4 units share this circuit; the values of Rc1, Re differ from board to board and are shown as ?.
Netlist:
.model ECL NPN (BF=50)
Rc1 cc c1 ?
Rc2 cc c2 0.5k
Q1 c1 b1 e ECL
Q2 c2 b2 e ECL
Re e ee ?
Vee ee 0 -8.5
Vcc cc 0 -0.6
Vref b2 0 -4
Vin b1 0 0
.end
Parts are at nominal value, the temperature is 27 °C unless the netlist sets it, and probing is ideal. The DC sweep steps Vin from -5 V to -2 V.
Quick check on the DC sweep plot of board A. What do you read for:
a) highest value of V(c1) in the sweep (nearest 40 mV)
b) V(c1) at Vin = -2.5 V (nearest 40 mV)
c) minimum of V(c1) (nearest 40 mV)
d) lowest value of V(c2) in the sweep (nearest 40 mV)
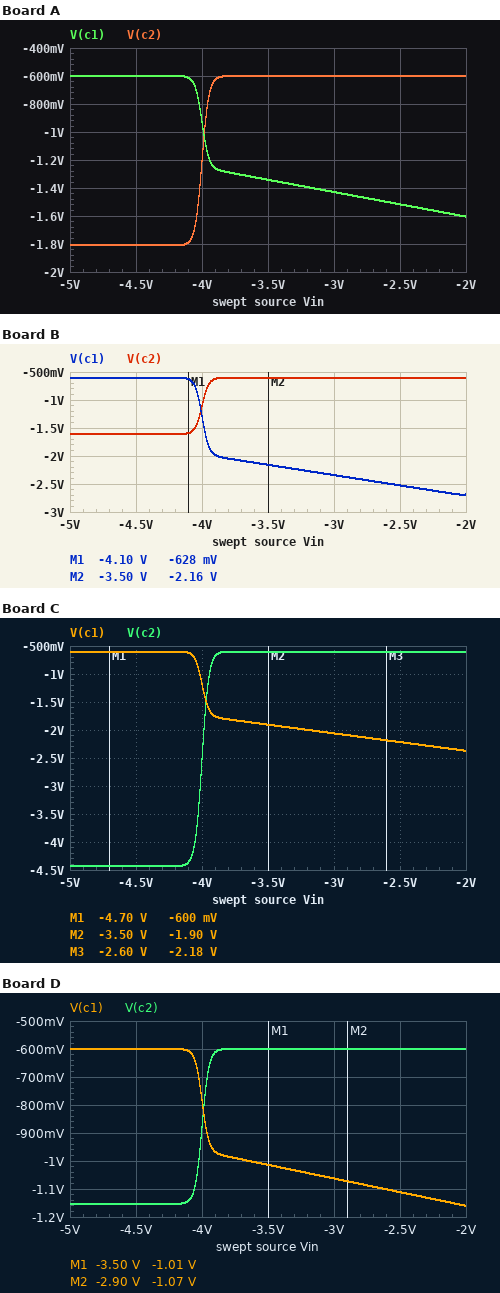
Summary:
-600 mV
-1.52 V
-1.60 V
-1.80 V
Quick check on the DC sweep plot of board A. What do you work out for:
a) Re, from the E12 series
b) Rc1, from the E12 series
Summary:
1.5 kΩ
270 Ω
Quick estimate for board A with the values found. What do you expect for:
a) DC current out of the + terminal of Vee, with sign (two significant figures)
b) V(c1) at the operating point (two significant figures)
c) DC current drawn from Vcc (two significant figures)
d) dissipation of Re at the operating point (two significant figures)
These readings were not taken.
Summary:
-5.1 mA
-810 mV
780 µA
39 mW
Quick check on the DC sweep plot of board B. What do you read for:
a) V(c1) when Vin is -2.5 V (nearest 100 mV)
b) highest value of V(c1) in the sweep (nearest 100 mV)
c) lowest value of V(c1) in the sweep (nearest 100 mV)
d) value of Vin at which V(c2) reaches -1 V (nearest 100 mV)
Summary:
-2.5 V
-600 mV
-2.7 V
-4.0 V
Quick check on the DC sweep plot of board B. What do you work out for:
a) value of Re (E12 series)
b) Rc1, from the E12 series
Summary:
1.8 kΩ
680 Ω
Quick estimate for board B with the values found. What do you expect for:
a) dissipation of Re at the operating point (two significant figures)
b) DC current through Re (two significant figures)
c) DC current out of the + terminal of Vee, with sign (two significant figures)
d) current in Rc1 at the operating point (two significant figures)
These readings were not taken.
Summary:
33 mW
4.3 mA
-4.3 mA
310 µA
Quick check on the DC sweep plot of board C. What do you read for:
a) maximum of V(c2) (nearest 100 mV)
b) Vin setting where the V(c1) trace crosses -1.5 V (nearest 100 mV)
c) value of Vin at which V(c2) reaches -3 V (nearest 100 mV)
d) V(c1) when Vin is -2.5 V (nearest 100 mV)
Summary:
-600 mV
-4.0 V
-4.0 V
-2.2 V
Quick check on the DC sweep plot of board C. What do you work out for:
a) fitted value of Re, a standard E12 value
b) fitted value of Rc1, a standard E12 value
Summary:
470 Ω
150 Ω
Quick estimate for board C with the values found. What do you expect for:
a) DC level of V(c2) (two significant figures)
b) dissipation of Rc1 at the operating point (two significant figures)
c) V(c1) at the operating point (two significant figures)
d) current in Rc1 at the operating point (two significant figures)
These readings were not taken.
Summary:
-600 mV
390 µW
-840 mV
1.6 mA
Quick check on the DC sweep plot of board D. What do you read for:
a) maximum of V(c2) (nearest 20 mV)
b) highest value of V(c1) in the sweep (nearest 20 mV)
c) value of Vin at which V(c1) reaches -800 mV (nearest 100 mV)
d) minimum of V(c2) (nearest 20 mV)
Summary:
-600 mV
-600 mV
-4.0 V
-1.16 V
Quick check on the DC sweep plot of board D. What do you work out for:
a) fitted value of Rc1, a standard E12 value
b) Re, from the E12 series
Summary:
330 Ω
3.3 kΩ
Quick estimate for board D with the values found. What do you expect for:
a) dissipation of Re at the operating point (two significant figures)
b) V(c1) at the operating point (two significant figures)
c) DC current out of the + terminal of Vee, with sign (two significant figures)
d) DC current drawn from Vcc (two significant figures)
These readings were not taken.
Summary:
18 mW
-790 mV
-2.3 mA
570 µA
